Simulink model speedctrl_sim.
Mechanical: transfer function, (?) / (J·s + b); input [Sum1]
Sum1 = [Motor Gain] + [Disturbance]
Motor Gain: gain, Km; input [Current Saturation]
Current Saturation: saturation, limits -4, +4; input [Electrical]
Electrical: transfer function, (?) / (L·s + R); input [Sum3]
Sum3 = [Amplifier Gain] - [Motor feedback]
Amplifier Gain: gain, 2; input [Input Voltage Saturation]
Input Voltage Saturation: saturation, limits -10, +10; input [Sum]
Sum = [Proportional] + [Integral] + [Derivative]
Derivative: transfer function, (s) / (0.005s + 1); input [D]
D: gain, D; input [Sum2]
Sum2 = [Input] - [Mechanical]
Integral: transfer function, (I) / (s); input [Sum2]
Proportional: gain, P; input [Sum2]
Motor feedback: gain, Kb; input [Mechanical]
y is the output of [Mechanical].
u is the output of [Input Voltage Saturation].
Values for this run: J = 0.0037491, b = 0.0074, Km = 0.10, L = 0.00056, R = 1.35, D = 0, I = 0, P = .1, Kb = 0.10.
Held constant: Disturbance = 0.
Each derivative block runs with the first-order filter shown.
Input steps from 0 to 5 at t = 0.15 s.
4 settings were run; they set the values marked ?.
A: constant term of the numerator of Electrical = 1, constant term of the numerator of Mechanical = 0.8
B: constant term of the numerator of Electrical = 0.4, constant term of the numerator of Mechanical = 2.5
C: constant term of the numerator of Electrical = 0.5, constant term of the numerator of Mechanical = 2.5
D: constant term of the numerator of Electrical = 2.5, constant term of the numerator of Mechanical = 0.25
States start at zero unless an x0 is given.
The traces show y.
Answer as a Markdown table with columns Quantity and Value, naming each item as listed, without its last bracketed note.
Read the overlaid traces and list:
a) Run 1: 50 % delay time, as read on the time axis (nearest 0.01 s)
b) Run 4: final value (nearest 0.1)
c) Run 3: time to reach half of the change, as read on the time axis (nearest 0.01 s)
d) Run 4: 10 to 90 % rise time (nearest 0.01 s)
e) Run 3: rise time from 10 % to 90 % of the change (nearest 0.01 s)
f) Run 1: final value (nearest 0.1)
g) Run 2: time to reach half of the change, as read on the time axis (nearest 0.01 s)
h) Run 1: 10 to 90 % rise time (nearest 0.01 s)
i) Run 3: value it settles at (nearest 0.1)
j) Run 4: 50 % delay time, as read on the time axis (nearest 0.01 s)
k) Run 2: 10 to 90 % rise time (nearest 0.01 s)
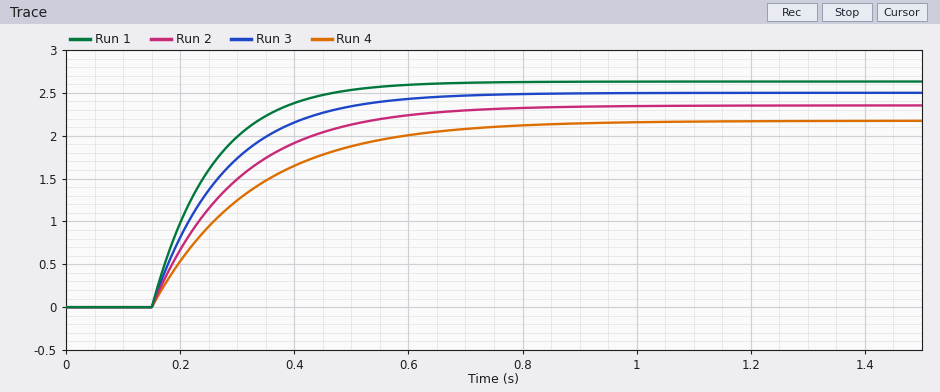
| Quantity | Value |
|---|---|
| Run 1: 50 % delay time, as read on the time axis | 0.22 s |
| Run 4: final value | 2.2 |
| Run 3: time to reach half of the change, as read on the time axis | 0.24 s |
| Run 4: 10 to 90 % rise time | 0.39 s |
| Run 3: rise time from 10 % to 90 % of the change | 0.28 s |
| Run 1: final value | 2.6 |
| Run 2: time to reach half of the change, as read on the time axis | 0.25 s |
| Run 1: 10 to 90 % rise time | 0.23 s |
| Run 3: value it settles at | 2.5 |
| Run 4: 50 % delay time, as read on the time axis | 0.27 s |
| Run 2: 10 to 90 % rise time | 0.33 s |
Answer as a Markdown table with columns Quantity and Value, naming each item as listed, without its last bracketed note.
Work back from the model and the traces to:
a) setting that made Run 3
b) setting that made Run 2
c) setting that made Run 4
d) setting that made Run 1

| Quantity | Value |
|---|---|
| setting that made Run 3 | B |
| setting that made Run 2 | A |
| setting that made Run 4 | D |
| setting that made Run 1 | C |
